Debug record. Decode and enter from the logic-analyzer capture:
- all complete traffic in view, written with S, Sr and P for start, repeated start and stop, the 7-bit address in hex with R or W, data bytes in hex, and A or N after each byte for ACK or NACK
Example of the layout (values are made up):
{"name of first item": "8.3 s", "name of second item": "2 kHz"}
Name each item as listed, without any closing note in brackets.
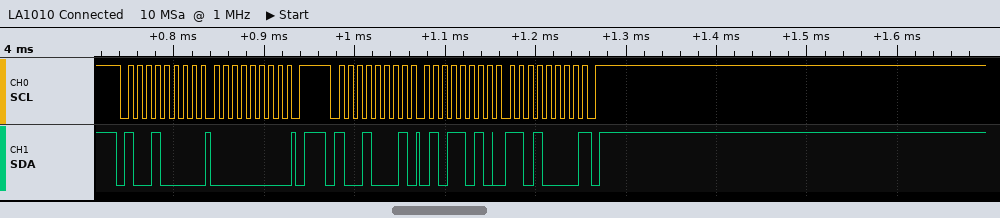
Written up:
{"all complete traffic in view, written with S, Sr and P for start, repeated start and stop, the 7-bit address in hex with R or W, data bytes in hex, and A or N after each byte for ACK or NACK": "S 48W A 00 A P S 48R A 5A A D0 N P"}
